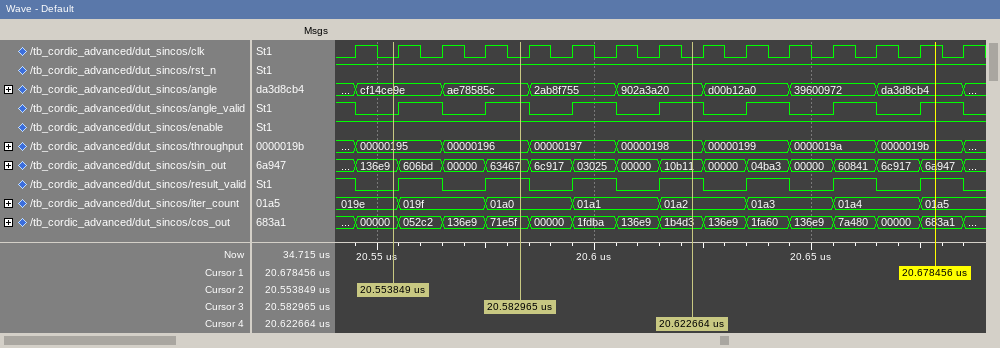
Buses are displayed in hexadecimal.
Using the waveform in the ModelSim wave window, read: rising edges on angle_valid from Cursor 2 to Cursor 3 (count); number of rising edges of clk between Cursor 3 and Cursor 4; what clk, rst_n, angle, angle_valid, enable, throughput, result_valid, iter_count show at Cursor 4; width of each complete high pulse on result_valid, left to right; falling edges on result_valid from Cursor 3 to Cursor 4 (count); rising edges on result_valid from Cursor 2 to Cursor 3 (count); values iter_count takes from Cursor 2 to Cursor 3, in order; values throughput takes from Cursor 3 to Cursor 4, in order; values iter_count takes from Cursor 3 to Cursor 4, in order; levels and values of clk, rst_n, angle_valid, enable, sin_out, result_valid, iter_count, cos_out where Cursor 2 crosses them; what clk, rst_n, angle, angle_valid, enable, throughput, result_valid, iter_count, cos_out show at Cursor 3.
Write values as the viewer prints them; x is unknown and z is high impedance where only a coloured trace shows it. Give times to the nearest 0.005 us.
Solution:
2
4
clk=0, rst_n=1, angle=902a3a20, angle_valid=1, enable=1, throughput=00000198, result_valid=1, iter_count=01a2
0.01 us, 0.01 us, 0.01 us, 0.01 us, 0.01 us, 0.01 us, 0.01 us
2
2
019e, 019f, 01a0
00000196, 00000197, 00000198
01a0, 01a1, 01a2
clk=0, rst_n=1, angle_valid=0, enable=1, sin_out=136e9, result_valid=0, iter_count=019e, cos_out=00000
clk=0, rst_n=1, angle=ae78585c, angle_valid=1, enable=1, throughput=00000196, result_valid=1, iter_count=01a0, cos_out=71e5f
